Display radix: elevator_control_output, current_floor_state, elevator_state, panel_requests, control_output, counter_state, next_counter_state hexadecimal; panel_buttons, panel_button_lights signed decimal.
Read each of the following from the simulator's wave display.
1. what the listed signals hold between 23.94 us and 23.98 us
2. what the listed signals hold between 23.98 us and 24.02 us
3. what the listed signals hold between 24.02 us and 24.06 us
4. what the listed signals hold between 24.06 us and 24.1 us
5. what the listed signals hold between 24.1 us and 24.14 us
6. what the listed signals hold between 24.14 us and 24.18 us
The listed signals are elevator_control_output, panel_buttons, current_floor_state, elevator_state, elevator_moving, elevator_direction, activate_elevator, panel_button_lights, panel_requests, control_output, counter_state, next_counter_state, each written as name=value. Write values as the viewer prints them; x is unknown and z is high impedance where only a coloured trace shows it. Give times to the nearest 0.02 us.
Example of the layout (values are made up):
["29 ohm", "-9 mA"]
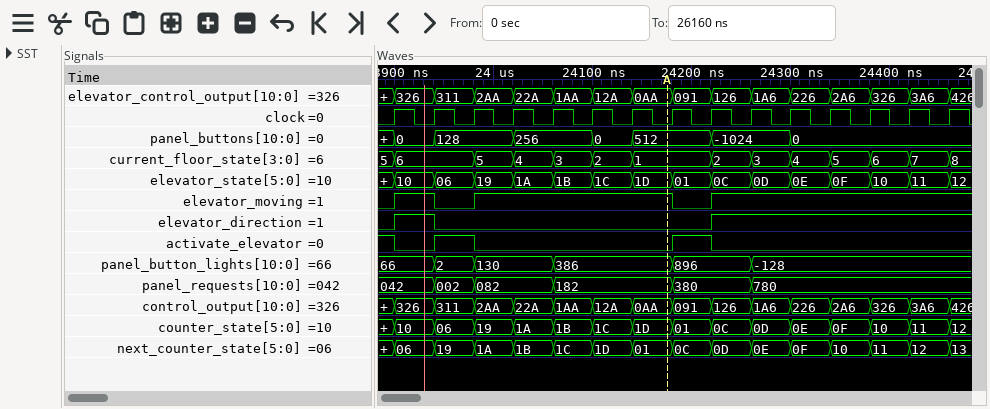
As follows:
["elevator_control_output=311, panel_buttons=128, current_floor_state=6, elevator_state=06, elevator_moving=0, elevator_direction=0, activate_elevator=1, panel_button_lights=2, panel_requests=002, control_output=311, counter_state=06, next_counter_state=19", "elevator_control_output=2AA, panel_buttons=128, current_floor_state=5, elevator_state=19, elevator_moving=1, elevator_direction=0, activate_elevator=0, panel_button_lights=130, panel_requests=082, control_output=2AA, counter_state=19, next_counter_state=1A", "elevator_control_output=22A, panel_buttons=256, current_floor_state=4, elevator_state=1A, elevator_moving=1, elevator_direction=0, activate_elevator=0, panel_button_lights=130, panel_requests=082, control_output=22A, counter_state=1A, next_counter_state=1B", "elevator_control_output=1AA, panel_buttons=256, current_floor_state=3, elevator_state=1B, elevator_moving=1, elevator_direction=0, activate_elevator=0, panel_button_lights=386, panel_requests=182, control_output=1AA, counter_state=1B, next_counter_state=1C", "elevator_control_output=12A, panel_buttons=0, current_floor_state=2, elevator_state=1C, elevator_moving=1, elevator_direction=0, activate_elevator=0, panel_button_lights=386, panel_requests=182, control_output=12A, counter_state=1C, next_counter_state=1D", "elevator_control_output=0AA, panel_buttons=512, current_floor_state=1, elevator_state=1D, elevator_moving=1, elevator_direction=0, activate_elevator=0, panel_button_lights=386, panel_requests=182, control_output=0AA, counter_state=1D, next_counter_state=01"]
